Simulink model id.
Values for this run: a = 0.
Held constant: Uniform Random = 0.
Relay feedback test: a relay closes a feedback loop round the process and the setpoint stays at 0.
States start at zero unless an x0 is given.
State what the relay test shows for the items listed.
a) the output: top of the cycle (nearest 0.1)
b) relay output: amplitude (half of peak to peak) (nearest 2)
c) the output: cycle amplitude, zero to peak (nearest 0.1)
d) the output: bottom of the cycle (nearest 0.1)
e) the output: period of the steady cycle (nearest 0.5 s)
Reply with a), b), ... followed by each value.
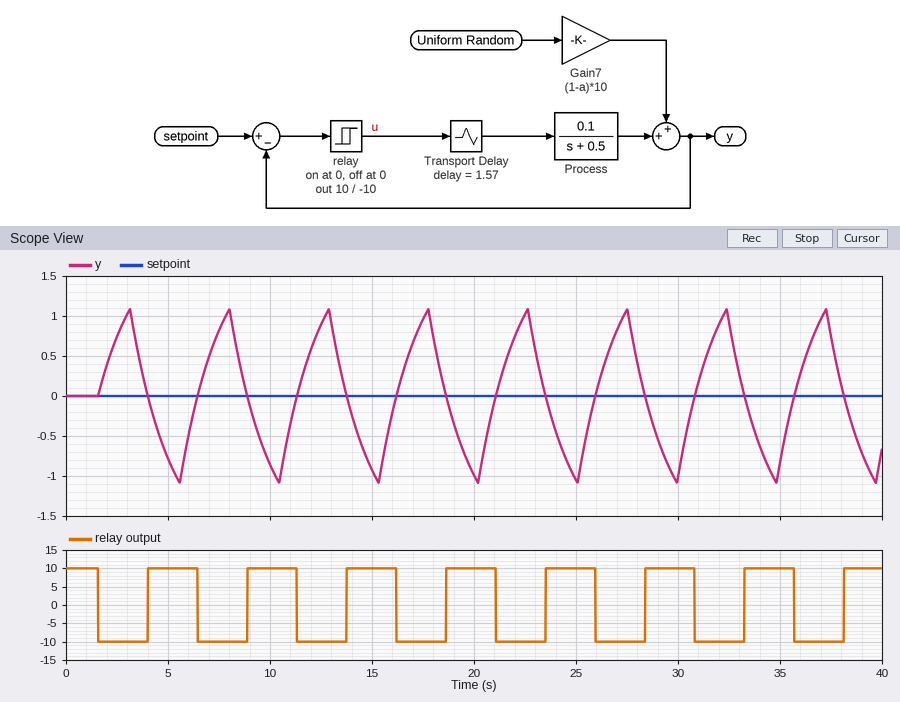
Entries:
a) 1.1
b) 10
c) 1.1
d) -1.1
e) 5.0 s
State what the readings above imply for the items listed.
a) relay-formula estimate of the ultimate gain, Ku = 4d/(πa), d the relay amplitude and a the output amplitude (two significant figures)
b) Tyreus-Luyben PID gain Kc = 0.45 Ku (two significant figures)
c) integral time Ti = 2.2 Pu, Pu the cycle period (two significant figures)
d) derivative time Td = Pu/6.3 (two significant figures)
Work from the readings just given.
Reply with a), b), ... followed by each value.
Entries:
a) 12
b) 5.4
c) 11 s
d) 0.79 s
